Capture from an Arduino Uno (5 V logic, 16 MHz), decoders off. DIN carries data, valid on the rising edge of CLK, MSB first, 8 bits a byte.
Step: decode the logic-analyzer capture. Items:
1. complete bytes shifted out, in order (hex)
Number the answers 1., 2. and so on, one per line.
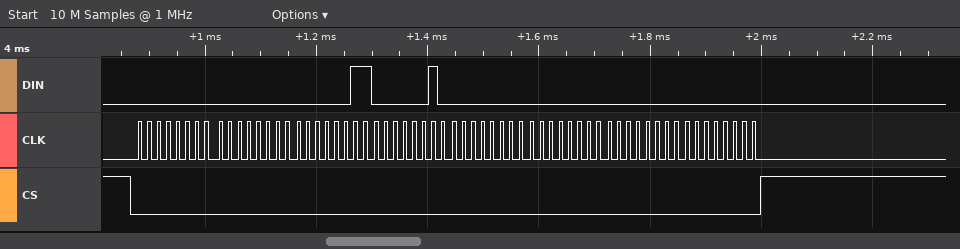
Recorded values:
1. 0x00 0x00 0x03 0x02 0x00 0x00 0x00 0x00
